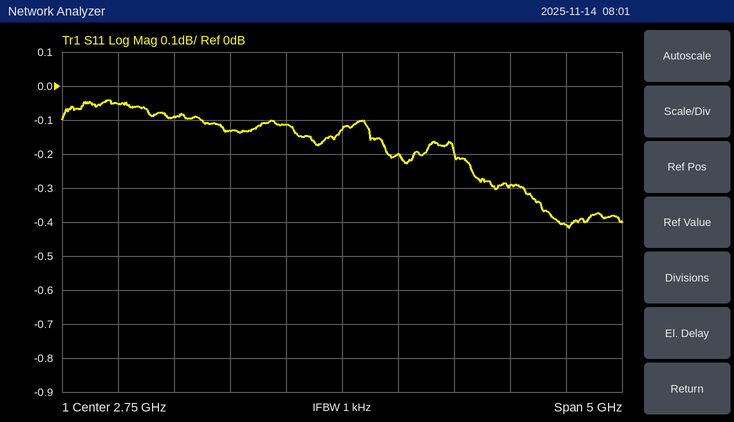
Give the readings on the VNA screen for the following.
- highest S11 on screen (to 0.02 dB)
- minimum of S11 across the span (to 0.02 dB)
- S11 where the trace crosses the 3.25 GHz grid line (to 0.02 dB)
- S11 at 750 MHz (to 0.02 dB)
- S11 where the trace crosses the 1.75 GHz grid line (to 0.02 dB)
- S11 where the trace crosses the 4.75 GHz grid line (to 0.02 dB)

-0.04 dB
-0.42 dB
-0.20 dB
-0.06 dB
-0.14 dB
-0.40 dB
